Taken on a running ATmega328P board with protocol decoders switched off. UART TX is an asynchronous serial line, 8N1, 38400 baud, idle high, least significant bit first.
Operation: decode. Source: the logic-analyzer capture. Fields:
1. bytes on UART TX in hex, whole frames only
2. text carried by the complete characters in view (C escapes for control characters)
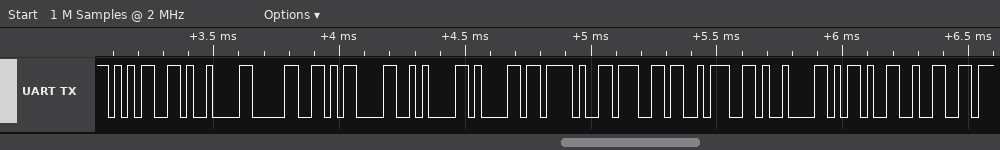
0x35 0x09 0x30 0x0D 0x0A 0x61 0x2F 0x67 0x3A 0x09 0x2D 0x32
"5\t0\r\na/g:\t-2"
